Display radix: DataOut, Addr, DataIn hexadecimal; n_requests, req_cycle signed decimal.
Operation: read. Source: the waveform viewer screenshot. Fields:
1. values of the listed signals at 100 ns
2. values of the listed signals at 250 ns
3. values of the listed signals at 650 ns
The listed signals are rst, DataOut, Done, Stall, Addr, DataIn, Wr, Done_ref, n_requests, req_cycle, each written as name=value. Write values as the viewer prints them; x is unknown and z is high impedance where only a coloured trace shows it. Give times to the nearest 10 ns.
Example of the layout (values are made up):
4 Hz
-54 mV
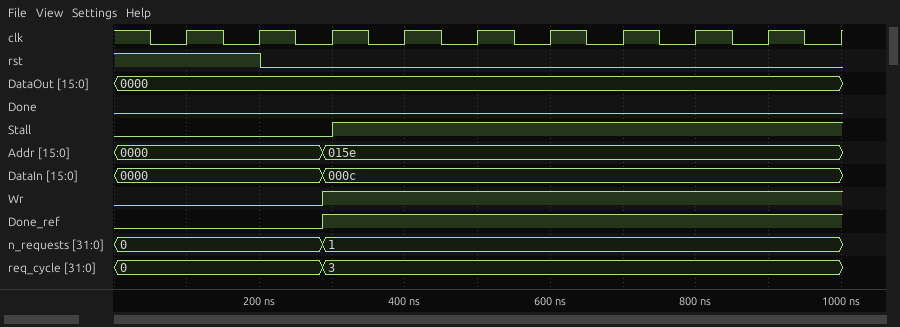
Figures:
rst=1, DataOut=0000, Done=0, Stall=0, Addr=0000, DataIn=0000, Wr=0, Done_ref=0, n_requests=0, req_cycle=0
rst=0, DataOut=0000, Done=0, Stall=0, Addr=0000, DataIn=0000, Wr=0, Done_ref=0, n_requests=0, req_cycle=0
rst=0, DataOut=0000, Done=0, Stall=1, Addr=015e, DataIn=000c, Wr=1, Done_ref=1, n_requests=1, req_cycle=3
